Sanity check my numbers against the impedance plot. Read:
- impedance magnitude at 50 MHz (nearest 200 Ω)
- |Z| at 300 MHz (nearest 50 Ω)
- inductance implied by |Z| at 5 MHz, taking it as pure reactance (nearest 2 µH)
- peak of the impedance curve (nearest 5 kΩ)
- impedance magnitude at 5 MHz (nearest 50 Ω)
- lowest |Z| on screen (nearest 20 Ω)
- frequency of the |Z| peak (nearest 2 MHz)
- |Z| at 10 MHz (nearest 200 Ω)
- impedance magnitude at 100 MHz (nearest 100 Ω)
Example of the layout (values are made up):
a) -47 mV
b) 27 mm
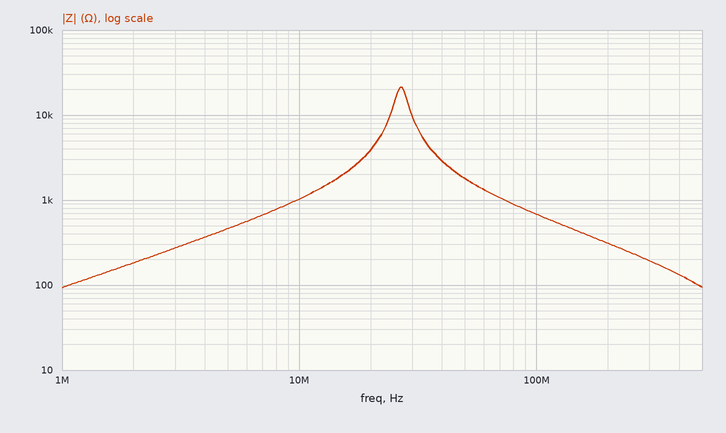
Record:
a) 1.8 kΩ
b) 200 Ω
c) 14 µH
d) 20 kΩ
e) 450 Ω
f) 100 Ω
g) 26 MHz
h) 1.0 kΩ
i) 700 Ω
